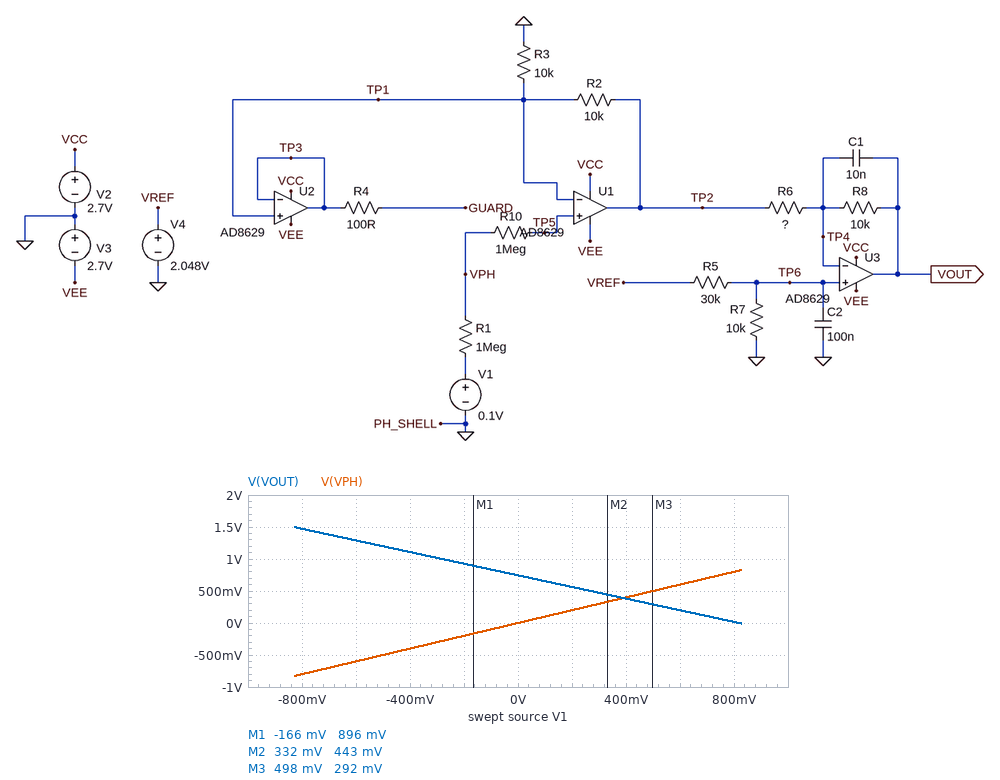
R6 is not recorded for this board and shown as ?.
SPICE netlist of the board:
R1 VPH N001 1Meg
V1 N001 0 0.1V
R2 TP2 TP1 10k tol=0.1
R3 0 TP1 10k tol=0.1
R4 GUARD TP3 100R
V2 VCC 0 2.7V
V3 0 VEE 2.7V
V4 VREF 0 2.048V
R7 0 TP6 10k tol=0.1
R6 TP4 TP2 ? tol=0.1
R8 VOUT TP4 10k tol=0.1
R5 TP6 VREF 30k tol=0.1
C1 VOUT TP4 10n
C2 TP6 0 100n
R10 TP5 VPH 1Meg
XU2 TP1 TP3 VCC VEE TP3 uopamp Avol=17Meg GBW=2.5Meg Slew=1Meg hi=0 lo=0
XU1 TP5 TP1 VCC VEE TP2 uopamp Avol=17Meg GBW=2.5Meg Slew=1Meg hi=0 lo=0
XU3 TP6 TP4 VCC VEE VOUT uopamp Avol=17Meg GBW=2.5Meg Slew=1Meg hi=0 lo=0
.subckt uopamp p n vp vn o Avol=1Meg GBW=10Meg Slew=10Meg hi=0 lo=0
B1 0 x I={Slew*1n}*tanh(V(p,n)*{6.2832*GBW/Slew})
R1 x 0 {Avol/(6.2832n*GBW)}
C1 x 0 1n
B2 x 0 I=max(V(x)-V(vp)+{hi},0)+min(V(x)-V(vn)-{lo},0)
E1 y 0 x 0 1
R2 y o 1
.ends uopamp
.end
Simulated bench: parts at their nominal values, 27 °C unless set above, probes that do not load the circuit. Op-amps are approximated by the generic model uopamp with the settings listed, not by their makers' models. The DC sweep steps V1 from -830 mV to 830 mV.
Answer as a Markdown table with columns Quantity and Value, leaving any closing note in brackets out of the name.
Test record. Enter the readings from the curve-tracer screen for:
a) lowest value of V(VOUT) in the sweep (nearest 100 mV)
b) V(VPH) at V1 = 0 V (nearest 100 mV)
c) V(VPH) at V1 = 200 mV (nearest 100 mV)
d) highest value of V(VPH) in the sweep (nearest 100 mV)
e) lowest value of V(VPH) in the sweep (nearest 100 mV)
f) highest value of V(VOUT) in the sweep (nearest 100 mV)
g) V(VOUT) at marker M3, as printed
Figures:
| Quantity | Value |
|---|---|
| lowest value of V(VOUT) in the sweep | 0 V |
| V(VPH) at V1 = 0 V | 0 V |
| V(VPH) at V1 = 200 mV | 200 mV |
| highest value of V(VPH) in the sweep | 800 mV |
| lowest value of V(VPH) in the sweep | -800 mV |
| highest value of V(VOUT) in the sweep | 1.5 V |
| V(VOUT) at marker M3, as printed | 292 mV |
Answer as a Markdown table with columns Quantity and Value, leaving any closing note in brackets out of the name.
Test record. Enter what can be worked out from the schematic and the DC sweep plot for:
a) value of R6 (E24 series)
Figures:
| Quantity | Value |
|---|---|
| value of R6 | 22 kΩ |
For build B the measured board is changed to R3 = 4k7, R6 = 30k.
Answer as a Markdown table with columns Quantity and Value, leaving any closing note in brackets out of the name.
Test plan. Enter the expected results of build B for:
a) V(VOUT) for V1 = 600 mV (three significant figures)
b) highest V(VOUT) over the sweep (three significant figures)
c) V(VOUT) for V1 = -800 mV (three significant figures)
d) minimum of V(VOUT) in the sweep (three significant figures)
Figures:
| Quantity | Value |
|---|---|
| V(VOUT) for V1 = 600 mV | 57.1 mV |
| highest V(VOUT) over the sweep | 1.55 V |
| V(VOUT) for V1 = -800 mV | 1.52 V |
| minimum of V(VOUT) in the sweep | -183 mV |
